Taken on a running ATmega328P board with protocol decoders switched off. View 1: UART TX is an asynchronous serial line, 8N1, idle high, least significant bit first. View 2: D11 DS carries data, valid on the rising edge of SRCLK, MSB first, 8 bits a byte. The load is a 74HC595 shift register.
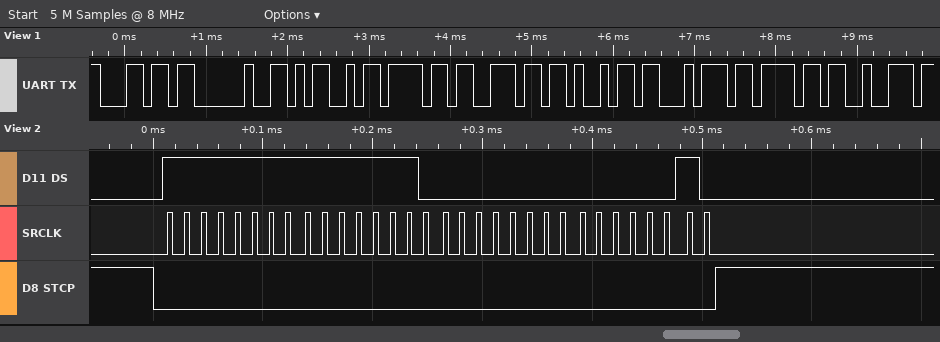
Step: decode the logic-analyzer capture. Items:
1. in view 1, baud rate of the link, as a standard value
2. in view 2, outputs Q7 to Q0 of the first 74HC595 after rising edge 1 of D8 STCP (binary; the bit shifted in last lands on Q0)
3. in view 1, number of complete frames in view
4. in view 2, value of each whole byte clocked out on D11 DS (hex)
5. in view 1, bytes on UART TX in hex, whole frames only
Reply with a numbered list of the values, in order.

1. 9600 baud
2. 00000010
3. 9
4. FF FE 00 02
5. 6C 20 4D 6F 6E 69 74 6F 72
